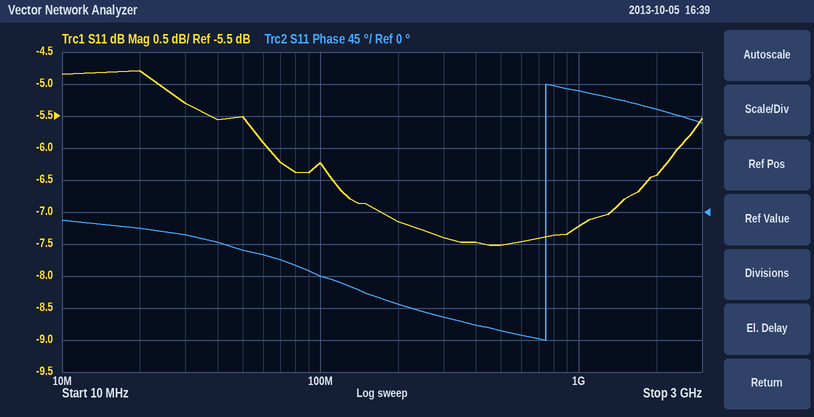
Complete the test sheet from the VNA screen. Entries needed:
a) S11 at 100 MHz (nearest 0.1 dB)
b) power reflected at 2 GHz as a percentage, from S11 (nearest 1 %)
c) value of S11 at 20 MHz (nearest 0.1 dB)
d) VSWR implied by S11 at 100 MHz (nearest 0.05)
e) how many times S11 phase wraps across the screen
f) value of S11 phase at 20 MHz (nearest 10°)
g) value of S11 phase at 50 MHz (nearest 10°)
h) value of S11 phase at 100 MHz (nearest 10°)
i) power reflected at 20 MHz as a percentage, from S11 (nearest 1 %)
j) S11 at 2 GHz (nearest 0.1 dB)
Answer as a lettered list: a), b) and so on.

a) -6.2 dB
b) 23 %
c) -4.8 dB
d) 2.90
e) 1
f) -20°
g) -50°
h) -90°
i) 33 %
j) -6.4 dB
